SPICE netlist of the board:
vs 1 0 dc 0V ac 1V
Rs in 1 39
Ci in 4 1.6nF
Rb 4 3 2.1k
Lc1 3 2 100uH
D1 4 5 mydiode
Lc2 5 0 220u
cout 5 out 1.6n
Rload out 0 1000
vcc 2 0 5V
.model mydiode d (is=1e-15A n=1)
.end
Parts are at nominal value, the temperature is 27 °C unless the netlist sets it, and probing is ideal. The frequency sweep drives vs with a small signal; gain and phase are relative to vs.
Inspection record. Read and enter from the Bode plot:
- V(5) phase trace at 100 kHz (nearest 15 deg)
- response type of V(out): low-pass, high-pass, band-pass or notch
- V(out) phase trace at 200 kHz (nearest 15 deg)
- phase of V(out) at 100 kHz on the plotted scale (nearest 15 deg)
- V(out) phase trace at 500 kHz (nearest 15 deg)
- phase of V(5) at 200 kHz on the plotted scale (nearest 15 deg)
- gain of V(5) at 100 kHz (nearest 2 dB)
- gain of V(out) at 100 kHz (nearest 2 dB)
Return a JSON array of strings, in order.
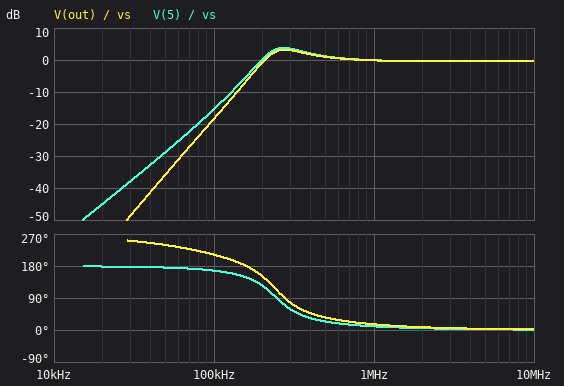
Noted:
["165 deg", "high-pass", "150 deg", "210 deg", "30 deg", "120 deg", "-16 dB", "-18 dB"]
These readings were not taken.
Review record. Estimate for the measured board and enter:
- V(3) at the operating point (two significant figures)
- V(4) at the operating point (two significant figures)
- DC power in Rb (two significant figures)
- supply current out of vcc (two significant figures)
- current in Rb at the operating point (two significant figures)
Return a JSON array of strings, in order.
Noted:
["5.0 V", "730 mV", "8.7 mW", "2.0 mA", "2.0 mA"]
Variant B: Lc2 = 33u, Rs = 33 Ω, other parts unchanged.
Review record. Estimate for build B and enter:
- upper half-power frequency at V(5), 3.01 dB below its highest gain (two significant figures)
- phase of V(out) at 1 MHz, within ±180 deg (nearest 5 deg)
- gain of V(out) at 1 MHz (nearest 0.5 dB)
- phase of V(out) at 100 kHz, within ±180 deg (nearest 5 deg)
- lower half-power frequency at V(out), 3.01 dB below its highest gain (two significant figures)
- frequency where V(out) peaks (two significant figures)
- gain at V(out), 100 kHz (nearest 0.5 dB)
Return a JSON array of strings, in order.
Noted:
["1.1 MHz", "40 deg", "3.5 dB", "-140 deg", "580 kHz", "720 kHz", "-36.5 dB"]
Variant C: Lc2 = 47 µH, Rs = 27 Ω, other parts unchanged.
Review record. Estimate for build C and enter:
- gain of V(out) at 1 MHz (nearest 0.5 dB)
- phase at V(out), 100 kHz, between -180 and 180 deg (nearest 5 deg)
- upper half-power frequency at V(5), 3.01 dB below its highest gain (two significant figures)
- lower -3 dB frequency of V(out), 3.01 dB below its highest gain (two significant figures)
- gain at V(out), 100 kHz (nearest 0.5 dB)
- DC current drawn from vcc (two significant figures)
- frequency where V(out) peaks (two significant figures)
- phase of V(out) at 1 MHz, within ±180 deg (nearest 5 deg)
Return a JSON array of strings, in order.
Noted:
["2.5 dB", "-140 deg", "860 kHz", "490 kHz", "-33.0 dB", "2.0 mA", "600 kHz", "25 deg"]
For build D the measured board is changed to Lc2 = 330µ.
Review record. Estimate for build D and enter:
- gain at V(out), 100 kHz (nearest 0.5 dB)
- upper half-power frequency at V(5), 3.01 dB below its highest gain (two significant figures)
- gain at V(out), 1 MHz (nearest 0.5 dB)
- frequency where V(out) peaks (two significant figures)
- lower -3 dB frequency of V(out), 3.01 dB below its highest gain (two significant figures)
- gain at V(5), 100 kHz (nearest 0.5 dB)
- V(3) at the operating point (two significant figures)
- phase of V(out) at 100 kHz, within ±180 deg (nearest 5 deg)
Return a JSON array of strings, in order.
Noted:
["-14.0 dB", "850 kHz", "-0.5 dB", "230 kHz", "170 kHz", "-11.0 dB", "5.0 V", "-155 deg"]
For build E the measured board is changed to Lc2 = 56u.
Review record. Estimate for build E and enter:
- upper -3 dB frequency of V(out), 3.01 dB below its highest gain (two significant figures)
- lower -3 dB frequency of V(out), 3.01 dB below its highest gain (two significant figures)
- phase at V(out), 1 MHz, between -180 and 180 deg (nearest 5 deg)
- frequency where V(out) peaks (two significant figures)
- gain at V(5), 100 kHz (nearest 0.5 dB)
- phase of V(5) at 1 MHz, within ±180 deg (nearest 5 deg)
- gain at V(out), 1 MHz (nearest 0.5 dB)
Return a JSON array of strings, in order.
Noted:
["880 kHz", "440 kHz", "25 deg", "550 kHz", "-28.5 dB", "20 deg", "1.5 dB"]
